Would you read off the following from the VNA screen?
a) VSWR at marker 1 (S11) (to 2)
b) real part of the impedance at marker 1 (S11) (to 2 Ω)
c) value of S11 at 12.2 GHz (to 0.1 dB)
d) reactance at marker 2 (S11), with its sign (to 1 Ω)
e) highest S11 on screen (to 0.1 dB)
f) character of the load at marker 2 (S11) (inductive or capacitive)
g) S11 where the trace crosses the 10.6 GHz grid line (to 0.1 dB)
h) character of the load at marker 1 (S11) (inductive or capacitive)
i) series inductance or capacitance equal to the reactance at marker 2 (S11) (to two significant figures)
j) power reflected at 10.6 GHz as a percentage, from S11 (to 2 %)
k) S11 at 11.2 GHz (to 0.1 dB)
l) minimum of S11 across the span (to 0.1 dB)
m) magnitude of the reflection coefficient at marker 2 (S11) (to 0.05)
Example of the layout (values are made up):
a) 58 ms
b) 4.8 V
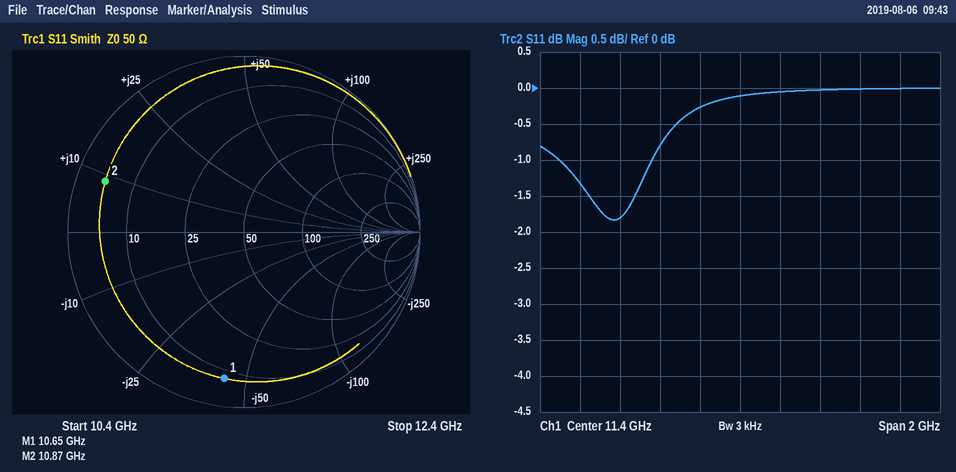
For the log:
a) 12
b) 8 Ω
c) 0.0 dB
d) +9 Ω
e) 0.0 dB
f) inductive
g) -1.3 dB
h) capacitive
i) 130 pH
j) 74 %
k) -0.3 dB
l) -1.8 dB
m) 0.85
